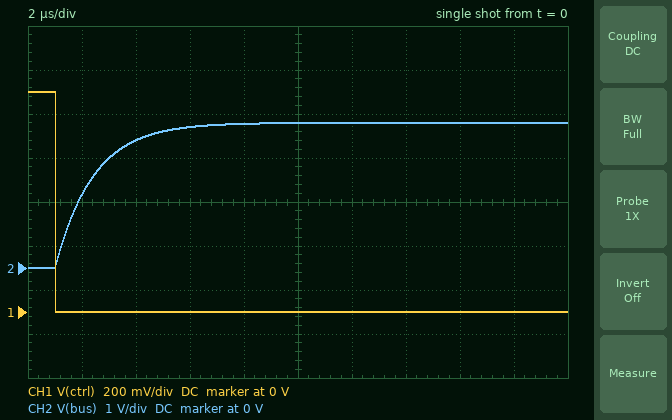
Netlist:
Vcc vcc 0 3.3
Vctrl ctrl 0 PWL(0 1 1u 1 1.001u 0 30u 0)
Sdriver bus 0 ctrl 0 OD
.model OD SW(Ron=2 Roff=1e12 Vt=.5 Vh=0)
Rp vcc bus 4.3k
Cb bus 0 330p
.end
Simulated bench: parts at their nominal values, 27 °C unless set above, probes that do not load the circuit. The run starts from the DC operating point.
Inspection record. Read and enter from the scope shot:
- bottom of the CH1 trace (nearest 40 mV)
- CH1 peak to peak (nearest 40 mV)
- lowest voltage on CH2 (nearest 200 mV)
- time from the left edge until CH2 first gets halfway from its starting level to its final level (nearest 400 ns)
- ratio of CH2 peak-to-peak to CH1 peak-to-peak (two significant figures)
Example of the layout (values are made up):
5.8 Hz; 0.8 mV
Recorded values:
0 V; 1.00 V; 0 V; 2.0 µs; 3.3
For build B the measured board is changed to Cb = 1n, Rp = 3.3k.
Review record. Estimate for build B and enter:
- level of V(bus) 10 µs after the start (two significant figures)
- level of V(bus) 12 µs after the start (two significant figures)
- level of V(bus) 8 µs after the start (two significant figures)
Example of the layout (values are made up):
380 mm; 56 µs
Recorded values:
3.1 V; 3.2 V; 2.9 V
